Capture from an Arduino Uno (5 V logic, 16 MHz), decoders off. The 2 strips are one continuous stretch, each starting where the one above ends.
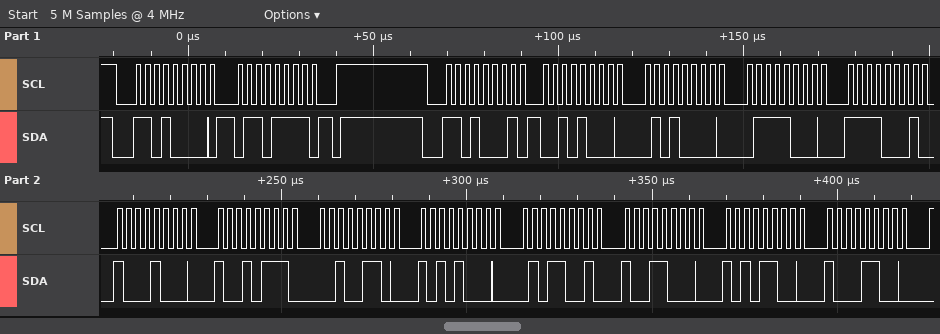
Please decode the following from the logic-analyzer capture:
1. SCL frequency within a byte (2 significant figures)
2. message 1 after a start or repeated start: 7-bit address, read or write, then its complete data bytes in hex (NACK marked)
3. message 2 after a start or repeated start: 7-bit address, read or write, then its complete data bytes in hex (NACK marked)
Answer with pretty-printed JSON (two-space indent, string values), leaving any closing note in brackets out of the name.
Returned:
{
  "SCL frequency within a byte": "400 kHz",
  "message 1 after a start or repeated start: 7-bit address, read or write, then its complete data bytes in hex": "0x68 write: 6F",
  "message 2 after a start or repeated start: 7-bit address, read or write, then its complete data bytes in hex": "0x68 read: 28 50 78 F1 88 97 26 A8 59 98 AC 8C"
}
